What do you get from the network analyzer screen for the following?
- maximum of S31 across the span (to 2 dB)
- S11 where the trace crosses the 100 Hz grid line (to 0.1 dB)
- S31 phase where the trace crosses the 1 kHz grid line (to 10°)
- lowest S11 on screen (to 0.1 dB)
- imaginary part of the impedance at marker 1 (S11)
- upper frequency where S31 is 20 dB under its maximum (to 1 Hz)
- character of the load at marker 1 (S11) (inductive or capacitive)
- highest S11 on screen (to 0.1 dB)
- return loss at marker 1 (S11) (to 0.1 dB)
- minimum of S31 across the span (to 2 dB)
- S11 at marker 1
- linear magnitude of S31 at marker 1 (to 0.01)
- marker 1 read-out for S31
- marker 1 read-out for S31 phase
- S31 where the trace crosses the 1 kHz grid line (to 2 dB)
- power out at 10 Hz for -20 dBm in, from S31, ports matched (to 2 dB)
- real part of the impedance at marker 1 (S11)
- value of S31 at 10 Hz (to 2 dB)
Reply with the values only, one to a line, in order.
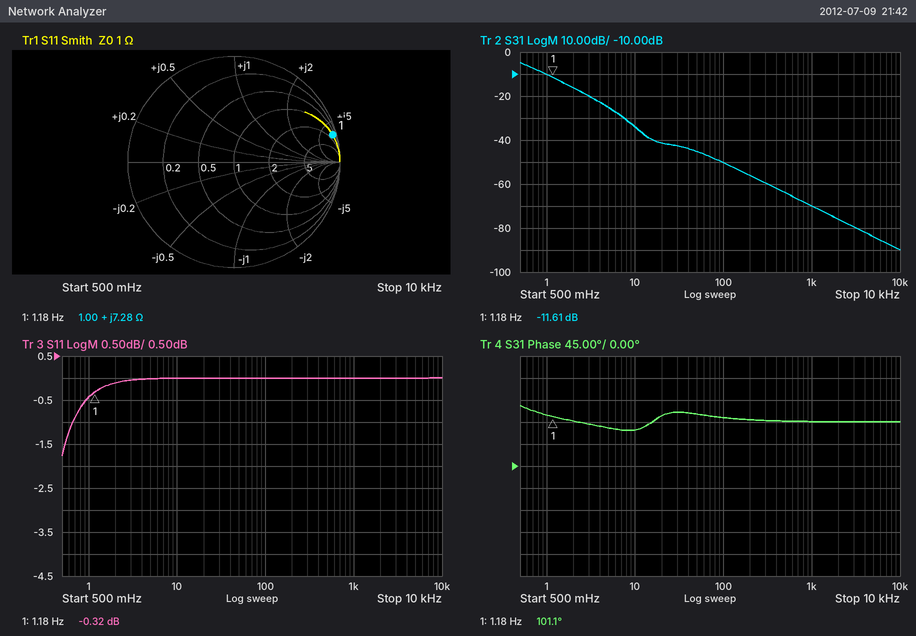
-4 dB
0.0 dB
90°
-1.8 dB
+7.28 Ω
5 Hz
inductive
0.0 dB
0.3 dB
-90 dB
-0.32 dB
0.26
-11.61 dB
101.1°
-70 dB
-54 dBm
1.00 Ω
-34 dB
